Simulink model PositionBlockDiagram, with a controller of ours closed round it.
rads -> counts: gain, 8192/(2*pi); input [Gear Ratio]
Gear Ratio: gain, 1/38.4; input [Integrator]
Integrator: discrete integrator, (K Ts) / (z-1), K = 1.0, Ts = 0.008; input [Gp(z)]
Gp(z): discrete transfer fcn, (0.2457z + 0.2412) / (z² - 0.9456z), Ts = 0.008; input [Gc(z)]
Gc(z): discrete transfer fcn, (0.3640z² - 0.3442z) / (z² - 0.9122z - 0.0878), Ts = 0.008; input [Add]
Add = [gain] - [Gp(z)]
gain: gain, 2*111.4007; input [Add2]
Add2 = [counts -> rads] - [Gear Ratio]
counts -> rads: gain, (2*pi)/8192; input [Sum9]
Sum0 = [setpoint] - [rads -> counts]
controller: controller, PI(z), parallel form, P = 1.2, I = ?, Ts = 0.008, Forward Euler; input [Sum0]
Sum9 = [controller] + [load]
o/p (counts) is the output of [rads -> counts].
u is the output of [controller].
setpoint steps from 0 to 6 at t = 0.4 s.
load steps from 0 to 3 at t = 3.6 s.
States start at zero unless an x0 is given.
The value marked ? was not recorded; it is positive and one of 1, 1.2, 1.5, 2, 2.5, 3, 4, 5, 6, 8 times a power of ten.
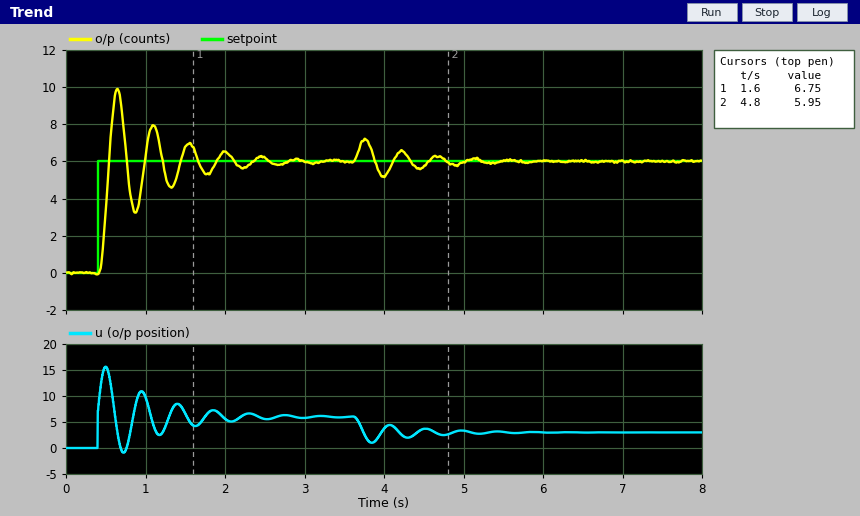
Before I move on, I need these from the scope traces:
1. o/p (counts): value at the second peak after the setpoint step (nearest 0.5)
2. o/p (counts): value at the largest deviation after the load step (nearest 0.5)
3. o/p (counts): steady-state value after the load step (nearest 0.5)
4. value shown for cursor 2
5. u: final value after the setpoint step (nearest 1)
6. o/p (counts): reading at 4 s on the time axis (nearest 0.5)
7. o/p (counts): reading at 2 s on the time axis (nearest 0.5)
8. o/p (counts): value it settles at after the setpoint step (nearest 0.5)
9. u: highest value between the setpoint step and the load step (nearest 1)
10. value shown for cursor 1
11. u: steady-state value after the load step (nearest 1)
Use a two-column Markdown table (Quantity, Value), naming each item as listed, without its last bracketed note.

| Quantity | Value |
|---|---|
| o/p (counts): value at the second peak after the setpoint step | 8.0 |
| o/p (counts): value at the largest deviation after the load step | 7.0 |
| o/p (counts): steady-state value after the load step | 6.0 |
| value shown for cursor 2 | 5.95 |
| u: final value after the setpoint step | 6 |
| o/p (counts): reading at 4 s on the time axis | 5.0 |
| o/p (counts): reading at 2 s on the time axis | 6.5 |
| o/p (counts): value it settles at after the setpoint step | 6.0 |
| u: highest value between the setpoint step and the load step | 16 |
| value shown for cursor 1 | 6.75 |
| u: steady-state value after the load step | 3 |
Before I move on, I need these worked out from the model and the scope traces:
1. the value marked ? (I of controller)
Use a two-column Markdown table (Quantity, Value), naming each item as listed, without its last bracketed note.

| Quantity | Value |
|---|---|
| the value marked ? | 25 |
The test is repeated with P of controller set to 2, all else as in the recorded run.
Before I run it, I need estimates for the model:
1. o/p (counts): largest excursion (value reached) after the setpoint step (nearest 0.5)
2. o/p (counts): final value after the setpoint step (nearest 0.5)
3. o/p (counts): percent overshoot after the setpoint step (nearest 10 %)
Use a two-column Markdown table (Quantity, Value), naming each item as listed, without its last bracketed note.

| Quantity | Value |
|---|---|
| o/p (counts): largest excursion (value reached) after the setpoint step | 9.0 |
| o/p (counts): final value after the setpoint step | 6.0 |
| o/p (counts): percent overshoot after the setpoint step | 50 % |
